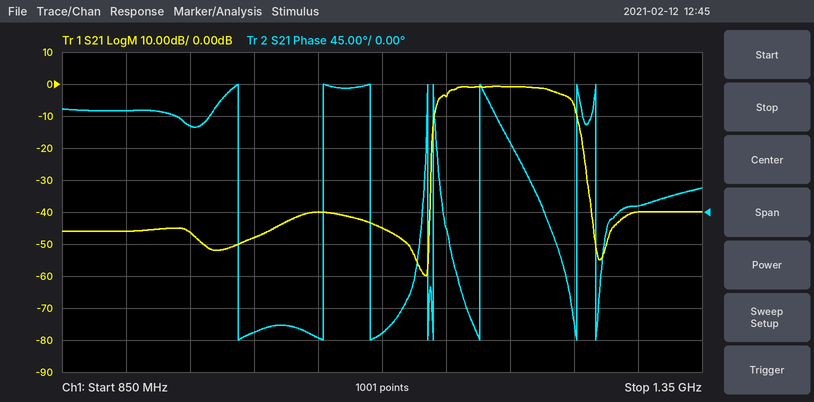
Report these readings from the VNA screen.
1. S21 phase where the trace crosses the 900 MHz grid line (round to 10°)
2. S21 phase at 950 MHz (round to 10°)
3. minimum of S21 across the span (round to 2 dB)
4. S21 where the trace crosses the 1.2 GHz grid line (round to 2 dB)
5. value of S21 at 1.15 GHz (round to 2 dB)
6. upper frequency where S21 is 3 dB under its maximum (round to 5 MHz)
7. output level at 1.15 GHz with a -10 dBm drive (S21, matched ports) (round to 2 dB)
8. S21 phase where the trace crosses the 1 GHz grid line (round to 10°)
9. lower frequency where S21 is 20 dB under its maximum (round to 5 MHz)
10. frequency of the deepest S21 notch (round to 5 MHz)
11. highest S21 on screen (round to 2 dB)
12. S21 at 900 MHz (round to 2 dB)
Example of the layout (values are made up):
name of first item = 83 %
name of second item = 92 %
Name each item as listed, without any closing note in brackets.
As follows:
S21 phase where the trace crosses the 900 MHz grid line = 140°
S21 phase at 950 MHz = 120°
minimum of S21 across the span = -60 dB
S21 where the trace crosses the 1.2 GHz grid line = 0 dB
value of S21 at 1.15 GHz = -4 dB
upper frequency where S21 is 3 dB under its maximum = 1.245 GHz
output level at 1.15 GHz with a -10 dBm drive (S21, matched ports) = -14 dBm
S21 phase where the trace crosses the 1 GHz grid line = -170°
lower frequency where S21 is 20 dB under its maximum = 1.140 GHz
frequency of the deepest S21 notch = 1.135 GHz
highest S21 on screen = 0 dB
S21 at 900 MHz = -46 dB
